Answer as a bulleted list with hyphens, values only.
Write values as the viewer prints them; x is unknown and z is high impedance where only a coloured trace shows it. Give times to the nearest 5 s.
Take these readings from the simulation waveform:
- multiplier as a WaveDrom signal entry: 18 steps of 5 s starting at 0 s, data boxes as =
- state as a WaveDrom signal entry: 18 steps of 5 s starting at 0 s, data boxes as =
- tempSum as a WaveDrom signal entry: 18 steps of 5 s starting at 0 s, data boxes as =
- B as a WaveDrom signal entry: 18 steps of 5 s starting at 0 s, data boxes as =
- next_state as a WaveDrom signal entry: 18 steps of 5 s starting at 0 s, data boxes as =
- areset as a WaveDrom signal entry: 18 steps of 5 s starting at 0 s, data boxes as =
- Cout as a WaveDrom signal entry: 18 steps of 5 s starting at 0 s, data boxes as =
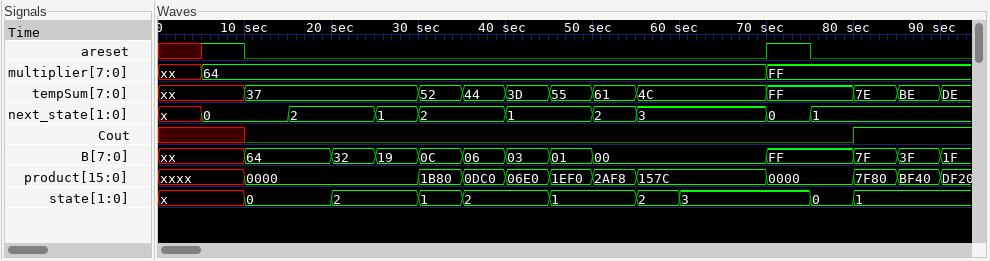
- {name: 'multiplier', wave: 'x=............=...', data: '64 FF'}
- {name: 'state', wave: 'x.=.=.==.=.==..==.', data: '0 2 1 2 1 2 3 0 1'}
- {name: 'tempSum', wave: 'x.=...======..=.==', data: '37 52 44 3D 55 61 4C FF 7E BE'}
- {name: 'B', wave: 'x.=.=======...=.==', data: '64 32 19 0C 06 03 01 00 FF 7F 3F'}
- {name: 'next_state', wave: 'x=.=.==.=.==..==..', data: '0 2 1 2 1 2 3 0 1'}
- {name: 'areset', wave: 'x10...........10..'}
- {name: 'Cout', wave: 'x.0.............1.'}
